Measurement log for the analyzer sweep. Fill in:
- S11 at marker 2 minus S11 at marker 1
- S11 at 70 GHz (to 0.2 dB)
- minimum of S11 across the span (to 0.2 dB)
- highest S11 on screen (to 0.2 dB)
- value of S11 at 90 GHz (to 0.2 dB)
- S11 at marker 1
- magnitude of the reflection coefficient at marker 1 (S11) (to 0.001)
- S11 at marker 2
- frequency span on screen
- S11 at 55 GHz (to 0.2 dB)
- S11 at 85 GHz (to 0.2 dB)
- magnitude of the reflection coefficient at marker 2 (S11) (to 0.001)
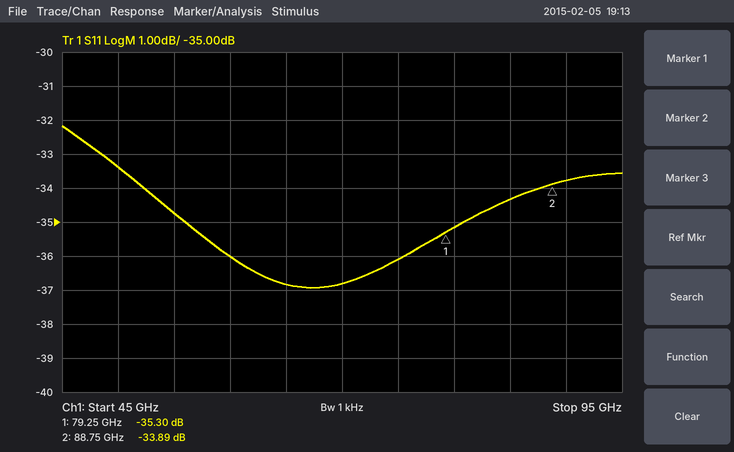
1.41 dB
-36.8 dB
-37.0 dB
-32.2 dB
-33.8 dB
-35.30 dB
0.017
-33.89 dB
50 GHz
-34.8 dB
-34.4 dB
0.020
